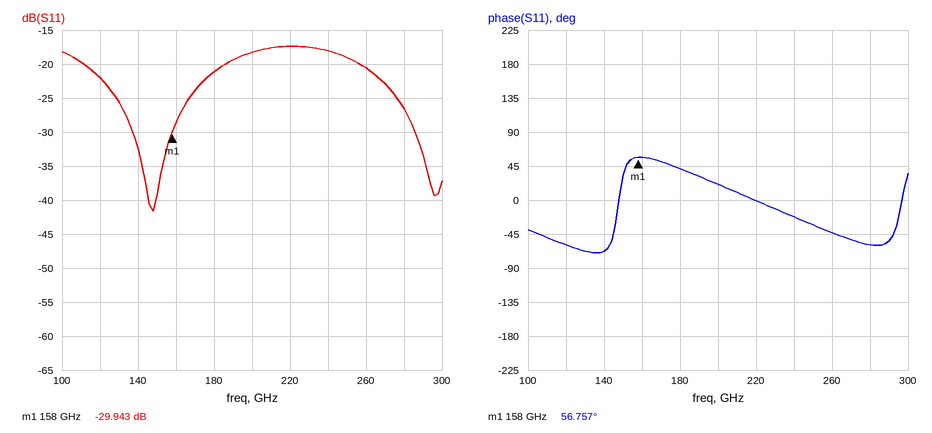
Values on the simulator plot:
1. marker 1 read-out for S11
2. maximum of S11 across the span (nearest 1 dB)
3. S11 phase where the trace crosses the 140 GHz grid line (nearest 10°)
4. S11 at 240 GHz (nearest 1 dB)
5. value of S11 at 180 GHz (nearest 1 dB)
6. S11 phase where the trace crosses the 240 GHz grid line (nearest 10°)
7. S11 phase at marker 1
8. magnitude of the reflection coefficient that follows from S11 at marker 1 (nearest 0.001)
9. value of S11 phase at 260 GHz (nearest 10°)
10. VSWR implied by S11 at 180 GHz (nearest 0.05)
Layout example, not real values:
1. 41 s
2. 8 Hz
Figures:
1. -29.943 dB
2. -17 dB
3. -70°
4. -18 dB
5. -21 dB
6. -20°
7. 56.757°
8. 0.032
9. -40°
10. 1.20
